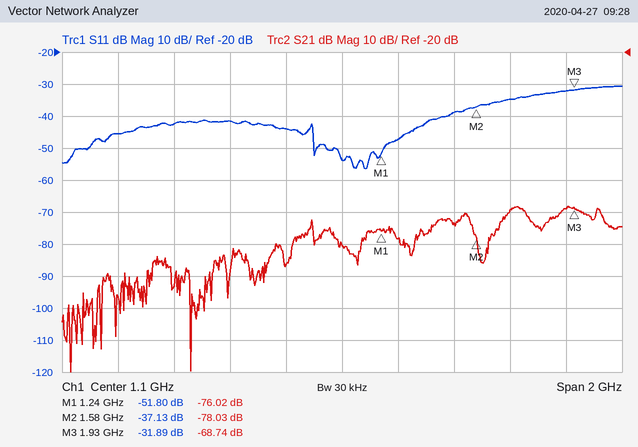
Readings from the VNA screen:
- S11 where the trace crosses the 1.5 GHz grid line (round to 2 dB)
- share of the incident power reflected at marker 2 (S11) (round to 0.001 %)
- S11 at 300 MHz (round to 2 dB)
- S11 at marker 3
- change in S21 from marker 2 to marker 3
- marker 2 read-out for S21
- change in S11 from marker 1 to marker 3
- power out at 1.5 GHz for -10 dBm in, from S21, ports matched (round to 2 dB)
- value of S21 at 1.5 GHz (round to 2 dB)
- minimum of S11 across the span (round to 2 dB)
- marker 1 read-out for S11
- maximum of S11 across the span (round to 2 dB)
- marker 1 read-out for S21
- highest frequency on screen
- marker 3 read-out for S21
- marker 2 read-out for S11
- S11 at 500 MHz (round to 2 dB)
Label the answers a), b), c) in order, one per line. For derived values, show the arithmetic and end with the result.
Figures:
a) -38 dB
b) 10^(-37.13/10) ≈ 0.019 %
c) -46 dB
d) -31.89 dB
e) -68.74 − (-78.03) = 9.29 dB
f) -78.03 dB
g) -31.89 − (-51.8) = 19.91 dB
h) -10 dBm + (-74 dB) = -84 dBm
i) -74 dB
j) -56 dB
k) -51.80 dB
l) -30 dB
m) -76.02 dB
n) 2.1 GHz
o) -68.74 dB
p) -37.13 dB
q) -42 dB
